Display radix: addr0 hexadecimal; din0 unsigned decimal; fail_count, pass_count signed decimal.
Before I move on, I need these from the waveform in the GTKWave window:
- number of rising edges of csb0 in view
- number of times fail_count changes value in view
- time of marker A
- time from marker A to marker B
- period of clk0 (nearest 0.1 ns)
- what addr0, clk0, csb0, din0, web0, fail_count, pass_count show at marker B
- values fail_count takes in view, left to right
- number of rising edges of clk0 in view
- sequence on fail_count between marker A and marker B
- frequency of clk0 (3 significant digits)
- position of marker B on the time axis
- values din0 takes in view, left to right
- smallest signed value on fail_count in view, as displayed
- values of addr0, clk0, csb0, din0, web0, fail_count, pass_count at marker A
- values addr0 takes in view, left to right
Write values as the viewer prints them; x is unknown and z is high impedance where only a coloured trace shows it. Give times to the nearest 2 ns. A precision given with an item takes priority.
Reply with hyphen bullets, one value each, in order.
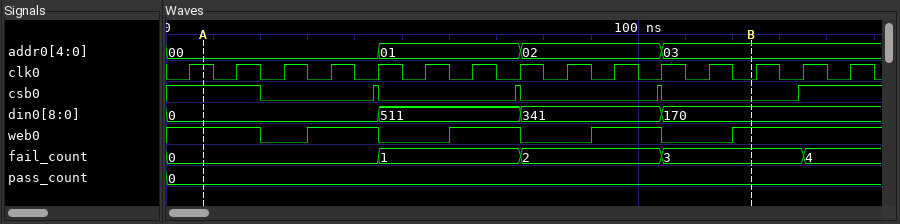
- 4
- 4
- 8 ns
- 116 ns
- 10 ns
- addr0=03, clk0=0, csb0=0, din0=170, web0=1, fail_count=3, pass_count=0
- 0, 1, 2, 3, 4
- 15
- 0, 1, 2, 3
- 100 MHz
- 124 ns
- 0, 511, 341, 170
- 0
- addr0=00, clk0=1, csb0=1, din0=0, web0=1, fail_count=0, pass_count=0
- 00, 01, 02, 03
